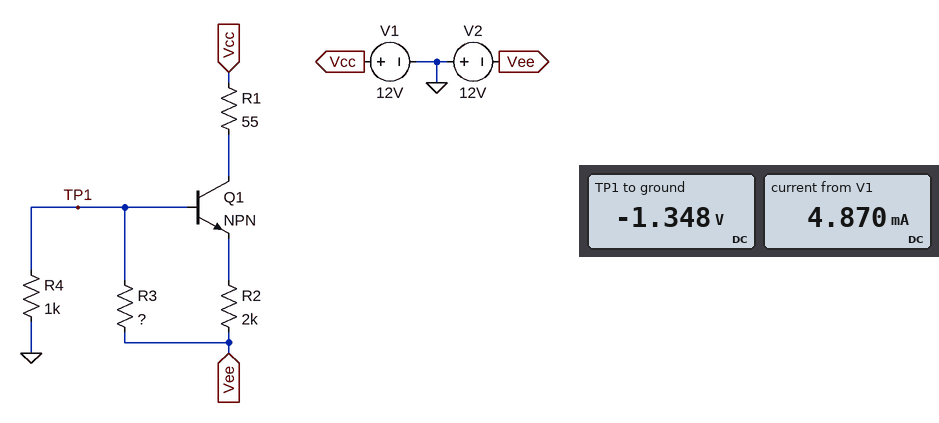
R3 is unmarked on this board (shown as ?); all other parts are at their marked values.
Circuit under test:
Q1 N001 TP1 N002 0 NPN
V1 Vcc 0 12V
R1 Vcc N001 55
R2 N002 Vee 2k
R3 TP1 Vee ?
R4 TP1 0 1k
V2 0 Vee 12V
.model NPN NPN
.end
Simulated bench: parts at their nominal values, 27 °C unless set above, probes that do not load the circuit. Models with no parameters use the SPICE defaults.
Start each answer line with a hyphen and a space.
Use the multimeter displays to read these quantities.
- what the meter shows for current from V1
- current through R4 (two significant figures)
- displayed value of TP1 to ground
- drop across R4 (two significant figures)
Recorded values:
- 4.870 mA
- 1.3 mA
- -1.348 V
- 1.3 V
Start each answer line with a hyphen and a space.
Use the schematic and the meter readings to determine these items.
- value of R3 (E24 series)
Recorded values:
- 8.2 kΩ
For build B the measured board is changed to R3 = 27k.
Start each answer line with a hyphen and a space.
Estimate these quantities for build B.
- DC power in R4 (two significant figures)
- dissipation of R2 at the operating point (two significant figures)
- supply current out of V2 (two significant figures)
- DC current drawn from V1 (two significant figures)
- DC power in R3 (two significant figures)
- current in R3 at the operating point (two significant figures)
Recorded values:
- 230 µW
- 57 mW
- 5.8 mA
- 5.3 mA
- 4.9 mW
- 430 µA
